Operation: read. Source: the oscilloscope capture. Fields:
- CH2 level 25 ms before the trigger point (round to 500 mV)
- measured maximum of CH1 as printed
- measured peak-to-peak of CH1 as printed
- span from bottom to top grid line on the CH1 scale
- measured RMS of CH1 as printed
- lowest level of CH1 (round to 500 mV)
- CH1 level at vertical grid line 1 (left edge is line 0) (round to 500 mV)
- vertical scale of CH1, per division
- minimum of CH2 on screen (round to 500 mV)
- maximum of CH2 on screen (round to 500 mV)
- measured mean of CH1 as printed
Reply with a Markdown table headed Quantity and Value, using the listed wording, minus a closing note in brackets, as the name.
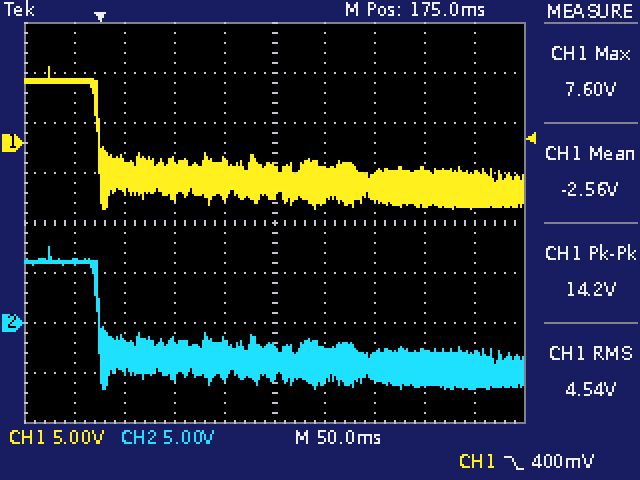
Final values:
| Quantity | Value |
|---|---|
| CH2 level 25 ms before the trigger point | 6.0 V |
| measured maximum of CH1 as printed | 7.60 V |
| measured peak-to-peak of CH1 as printed | 14.2 V |
| span from bottom to top grid line on the CH1 scale | 40 V |
| measured RMS of CH1 as printed | 4.54 V |
| lowest level of CH1 | -6.5 V |
| CH1 level at vertical grid line 1 (left edge is line 0) | 6.0 V |
| vertical scale of CH1, per division | 5 V |
| minimum of CH2 on screen | -6.5 V |
| maximum of CH2 on screen | 7.5 V |
| measured mean of CH1 as printed | -2.56 V |
